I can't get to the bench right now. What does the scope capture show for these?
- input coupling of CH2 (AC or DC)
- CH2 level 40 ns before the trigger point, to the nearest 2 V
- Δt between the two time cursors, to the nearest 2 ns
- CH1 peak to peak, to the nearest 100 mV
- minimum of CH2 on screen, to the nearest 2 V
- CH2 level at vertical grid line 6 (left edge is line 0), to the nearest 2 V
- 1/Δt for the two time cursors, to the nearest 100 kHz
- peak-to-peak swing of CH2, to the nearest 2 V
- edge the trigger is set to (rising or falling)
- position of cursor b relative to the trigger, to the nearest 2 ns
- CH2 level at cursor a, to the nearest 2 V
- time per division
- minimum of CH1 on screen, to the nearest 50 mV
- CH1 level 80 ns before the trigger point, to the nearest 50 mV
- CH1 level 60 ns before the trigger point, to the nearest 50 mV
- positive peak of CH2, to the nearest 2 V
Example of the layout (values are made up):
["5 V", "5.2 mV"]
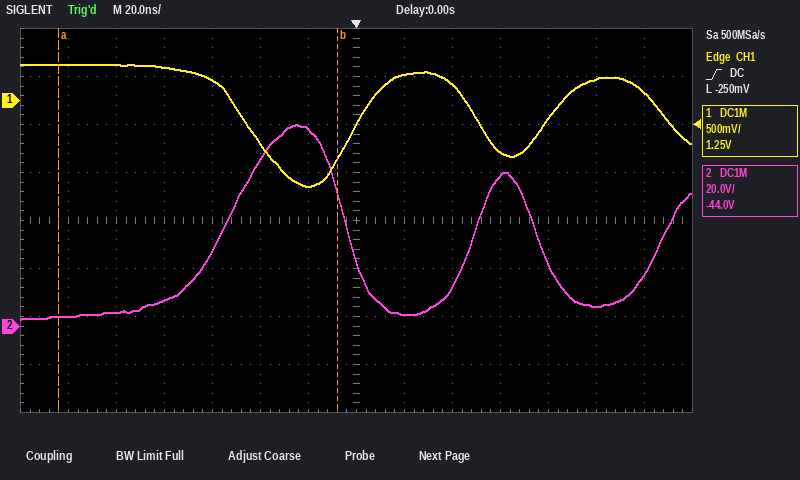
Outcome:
["DC", "70 V", "116 ns", "1.30 V", "2 V", "82 V", "8.6 MHz", "82 V", "rising", "-8 ns", "4 V", "20 ns", "-900 mV", "350 mV", "200 mV", "84 V"]
